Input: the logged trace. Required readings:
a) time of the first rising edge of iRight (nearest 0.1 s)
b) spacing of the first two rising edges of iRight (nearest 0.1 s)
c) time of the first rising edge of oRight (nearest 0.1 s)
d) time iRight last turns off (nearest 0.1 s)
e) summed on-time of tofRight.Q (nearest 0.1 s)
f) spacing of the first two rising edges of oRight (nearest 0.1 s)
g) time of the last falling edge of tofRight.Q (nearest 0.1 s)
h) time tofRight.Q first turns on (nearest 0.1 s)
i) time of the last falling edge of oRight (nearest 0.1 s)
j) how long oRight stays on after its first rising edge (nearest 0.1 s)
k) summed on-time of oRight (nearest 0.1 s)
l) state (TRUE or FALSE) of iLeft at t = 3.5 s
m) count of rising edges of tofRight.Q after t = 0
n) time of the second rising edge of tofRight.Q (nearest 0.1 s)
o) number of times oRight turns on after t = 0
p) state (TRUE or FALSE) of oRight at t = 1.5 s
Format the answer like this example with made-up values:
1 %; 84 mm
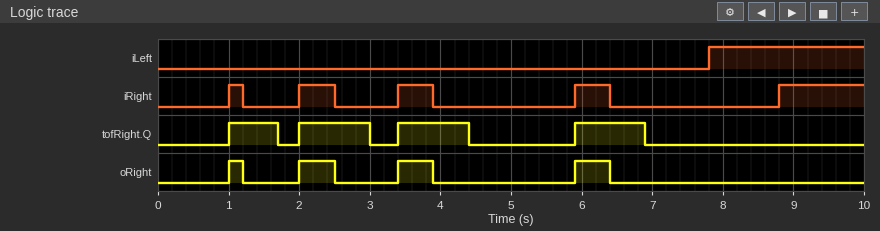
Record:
1.0 s; 1.0 s; 1.0 s; 6.4 s; 3.7 s; 1.0 s; 6.9 s; 1.0 s; 6.4 s; 0.2 s; 1.7 s; FALSE; 4; 2.0 s; 4; FALSE
